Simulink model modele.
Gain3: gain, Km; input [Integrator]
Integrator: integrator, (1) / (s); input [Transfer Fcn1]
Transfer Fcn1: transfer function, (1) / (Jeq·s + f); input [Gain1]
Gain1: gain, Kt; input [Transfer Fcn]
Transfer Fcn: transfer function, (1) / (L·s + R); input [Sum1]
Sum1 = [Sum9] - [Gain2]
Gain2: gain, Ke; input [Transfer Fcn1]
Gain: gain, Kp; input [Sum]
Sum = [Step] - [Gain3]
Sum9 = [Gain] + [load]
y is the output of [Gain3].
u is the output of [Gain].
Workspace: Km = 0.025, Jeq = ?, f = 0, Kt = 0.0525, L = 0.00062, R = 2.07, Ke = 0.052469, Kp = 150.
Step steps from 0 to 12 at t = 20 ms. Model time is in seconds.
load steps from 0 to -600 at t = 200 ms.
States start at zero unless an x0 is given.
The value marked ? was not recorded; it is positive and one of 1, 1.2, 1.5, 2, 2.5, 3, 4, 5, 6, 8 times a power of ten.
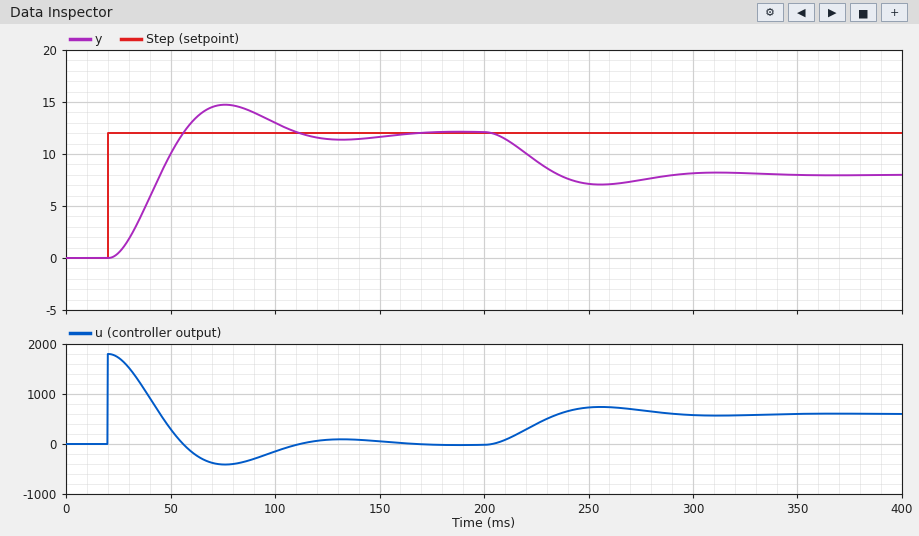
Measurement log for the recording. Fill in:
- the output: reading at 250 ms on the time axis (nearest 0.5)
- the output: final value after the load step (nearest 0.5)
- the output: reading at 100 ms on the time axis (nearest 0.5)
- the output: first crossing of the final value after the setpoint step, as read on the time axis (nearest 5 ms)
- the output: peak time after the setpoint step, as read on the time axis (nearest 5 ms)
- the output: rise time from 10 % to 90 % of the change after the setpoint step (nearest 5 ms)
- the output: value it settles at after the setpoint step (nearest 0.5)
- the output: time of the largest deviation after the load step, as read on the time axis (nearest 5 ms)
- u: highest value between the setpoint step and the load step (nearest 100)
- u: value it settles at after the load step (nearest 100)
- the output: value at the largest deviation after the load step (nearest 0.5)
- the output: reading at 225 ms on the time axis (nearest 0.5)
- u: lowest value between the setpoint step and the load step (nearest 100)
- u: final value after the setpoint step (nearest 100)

7.0
8.0
13.0
55 ms
75 ms
25 ms
12.0
255 ms
1800
600
7.0
9.5
-400
0
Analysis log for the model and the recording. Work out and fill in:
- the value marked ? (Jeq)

2.5e-05
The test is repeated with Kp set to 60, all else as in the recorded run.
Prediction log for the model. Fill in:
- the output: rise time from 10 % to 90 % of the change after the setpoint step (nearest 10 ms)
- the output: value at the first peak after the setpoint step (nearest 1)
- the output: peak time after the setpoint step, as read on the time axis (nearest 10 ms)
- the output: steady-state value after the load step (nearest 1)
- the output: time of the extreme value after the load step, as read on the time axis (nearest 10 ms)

50 ms
13
130 ms
2
310 ms
